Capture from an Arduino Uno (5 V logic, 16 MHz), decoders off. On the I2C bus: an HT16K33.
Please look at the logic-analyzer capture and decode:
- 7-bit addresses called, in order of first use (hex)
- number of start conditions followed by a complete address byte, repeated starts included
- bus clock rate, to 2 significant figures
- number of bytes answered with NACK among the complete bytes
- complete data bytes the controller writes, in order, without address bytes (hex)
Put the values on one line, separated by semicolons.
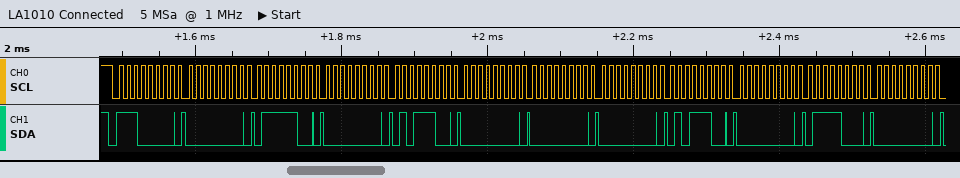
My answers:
0x70; 1; 100 kHz; 0; 00 7C 00 5C 00 00 00 5C 00 78 00
